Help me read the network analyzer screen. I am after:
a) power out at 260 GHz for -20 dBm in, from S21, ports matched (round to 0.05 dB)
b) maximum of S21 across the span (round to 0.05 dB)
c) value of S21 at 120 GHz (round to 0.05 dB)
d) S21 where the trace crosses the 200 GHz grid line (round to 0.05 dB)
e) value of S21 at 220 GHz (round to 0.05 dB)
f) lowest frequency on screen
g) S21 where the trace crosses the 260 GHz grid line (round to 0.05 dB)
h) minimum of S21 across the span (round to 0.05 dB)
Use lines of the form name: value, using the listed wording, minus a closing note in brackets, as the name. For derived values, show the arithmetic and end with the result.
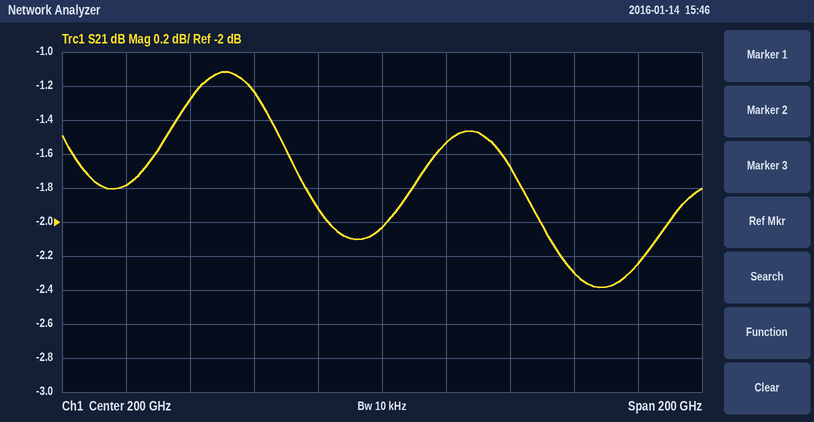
power out at 260 GHz for -20 dBm in, from S21, ports matched: -20 dBm + (-2.30 dB) = -22.30 dBm
maximum of S21 across the span: -1.10 dB
value of S21 at 120 GHz: -1.80 dB
S21 where the trace crosses the 200 GHz grid line: -2.05 dB
value of S21 at 220 GHz: -1.55 dB
lowest frequency on screen: 100 GHz
S21 where the trace crosses the 260 GHz grid line: -2.30 dB
minimum of S21 across the span: -2.40 dB
